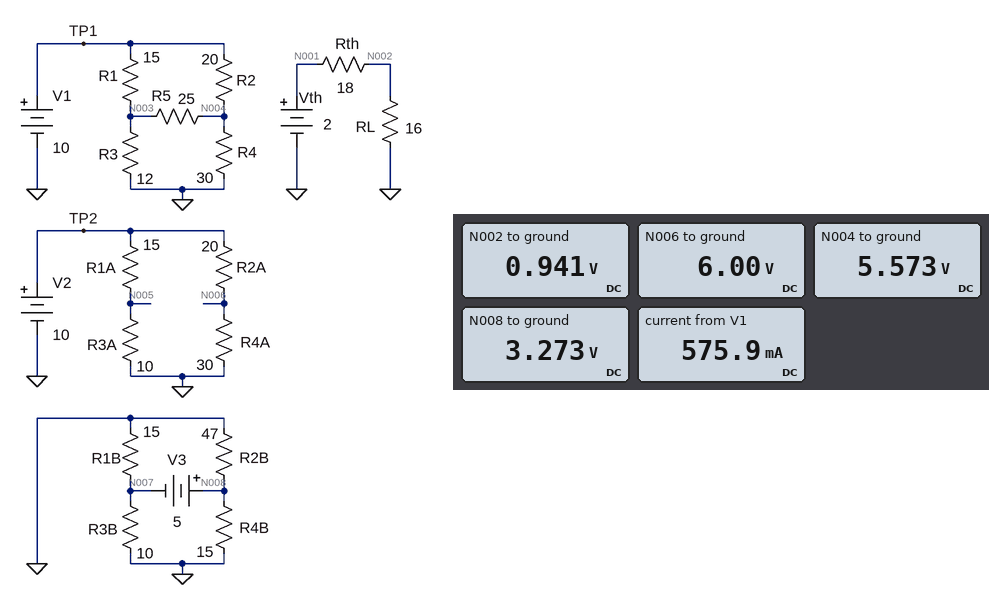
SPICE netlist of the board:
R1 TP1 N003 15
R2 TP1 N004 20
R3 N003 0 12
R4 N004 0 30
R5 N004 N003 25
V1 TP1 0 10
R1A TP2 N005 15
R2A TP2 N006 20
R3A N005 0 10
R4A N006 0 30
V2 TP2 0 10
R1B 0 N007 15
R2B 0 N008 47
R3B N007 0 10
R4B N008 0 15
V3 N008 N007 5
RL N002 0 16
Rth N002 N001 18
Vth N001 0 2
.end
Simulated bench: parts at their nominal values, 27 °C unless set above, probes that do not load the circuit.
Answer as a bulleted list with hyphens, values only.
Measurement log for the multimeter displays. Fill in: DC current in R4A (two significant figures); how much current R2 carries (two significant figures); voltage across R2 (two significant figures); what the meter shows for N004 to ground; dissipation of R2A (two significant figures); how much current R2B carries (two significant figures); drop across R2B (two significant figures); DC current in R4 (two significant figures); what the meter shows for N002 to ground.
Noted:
- 200 mA
- 220 mA
- 4.4 V
- 5.573 V
- 800 mW
- 70 mA
- 3.3 V
- 190 mA
- 0.941 V
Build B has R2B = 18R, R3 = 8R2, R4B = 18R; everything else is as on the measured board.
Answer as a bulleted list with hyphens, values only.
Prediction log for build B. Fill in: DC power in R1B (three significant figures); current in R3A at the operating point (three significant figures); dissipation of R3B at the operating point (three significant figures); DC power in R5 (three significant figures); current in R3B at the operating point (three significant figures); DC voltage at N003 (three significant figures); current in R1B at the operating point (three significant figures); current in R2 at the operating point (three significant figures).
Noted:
- 267 mW
- 400 mA
- 400 mW
- 84.9 mW
- 200 mA
- 3.84 V
- 133 mA
- 235 mA
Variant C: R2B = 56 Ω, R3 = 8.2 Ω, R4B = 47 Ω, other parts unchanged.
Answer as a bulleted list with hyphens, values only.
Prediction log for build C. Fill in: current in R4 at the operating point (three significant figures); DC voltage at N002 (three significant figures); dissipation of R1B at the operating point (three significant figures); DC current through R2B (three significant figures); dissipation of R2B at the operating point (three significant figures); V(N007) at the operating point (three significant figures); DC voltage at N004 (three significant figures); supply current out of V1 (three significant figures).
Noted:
- 177 mA
- 941 mV
- 60.3 mW
- 72.3 mA
- 293 mW
- -951 mV
- 5.30 V
- 645 mA
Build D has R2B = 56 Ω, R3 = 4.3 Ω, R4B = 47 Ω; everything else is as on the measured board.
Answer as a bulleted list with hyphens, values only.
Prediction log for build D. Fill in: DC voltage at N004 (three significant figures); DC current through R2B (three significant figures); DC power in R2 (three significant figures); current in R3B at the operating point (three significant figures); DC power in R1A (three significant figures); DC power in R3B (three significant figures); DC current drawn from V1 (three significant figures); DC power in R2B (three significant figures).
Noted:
- 4.88 V
- 72.3 mA
- 1.31 W
- 95.1 mA
- 2.40 W
- 90.4 mW
- 753 mA
- 293 mW
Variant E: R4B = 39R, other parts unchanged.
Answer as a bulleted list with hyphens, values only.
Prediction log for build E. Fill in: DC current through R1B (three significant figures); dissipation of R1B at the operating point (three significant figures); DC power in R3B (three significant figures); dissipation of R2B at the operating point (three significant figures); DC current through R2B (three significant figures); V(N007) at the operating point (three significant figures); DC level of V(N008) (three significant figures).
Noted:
- 73.2 mA
- 80.4 mW
- 121 mW
- 324 mW
- 83.0 mA
- -1.10 V
- 3.90 V
